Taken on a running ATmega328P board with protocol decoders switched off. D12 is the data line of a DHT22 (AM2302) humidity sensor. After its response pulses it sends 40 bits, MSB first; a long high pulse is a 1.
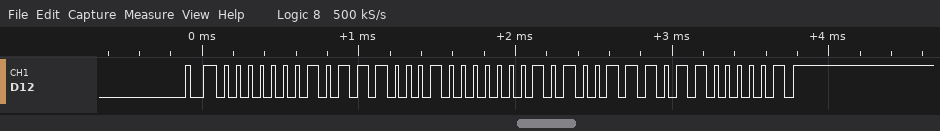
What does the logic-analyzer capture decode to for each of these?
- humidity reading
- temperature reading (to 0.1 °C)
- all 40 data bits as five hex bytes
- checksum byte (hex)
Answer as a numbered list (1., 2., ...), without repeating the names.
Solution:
1. 36.9 %
2. 33.4 °C
3. 01 71 01 4E C1
4. 0xC1
